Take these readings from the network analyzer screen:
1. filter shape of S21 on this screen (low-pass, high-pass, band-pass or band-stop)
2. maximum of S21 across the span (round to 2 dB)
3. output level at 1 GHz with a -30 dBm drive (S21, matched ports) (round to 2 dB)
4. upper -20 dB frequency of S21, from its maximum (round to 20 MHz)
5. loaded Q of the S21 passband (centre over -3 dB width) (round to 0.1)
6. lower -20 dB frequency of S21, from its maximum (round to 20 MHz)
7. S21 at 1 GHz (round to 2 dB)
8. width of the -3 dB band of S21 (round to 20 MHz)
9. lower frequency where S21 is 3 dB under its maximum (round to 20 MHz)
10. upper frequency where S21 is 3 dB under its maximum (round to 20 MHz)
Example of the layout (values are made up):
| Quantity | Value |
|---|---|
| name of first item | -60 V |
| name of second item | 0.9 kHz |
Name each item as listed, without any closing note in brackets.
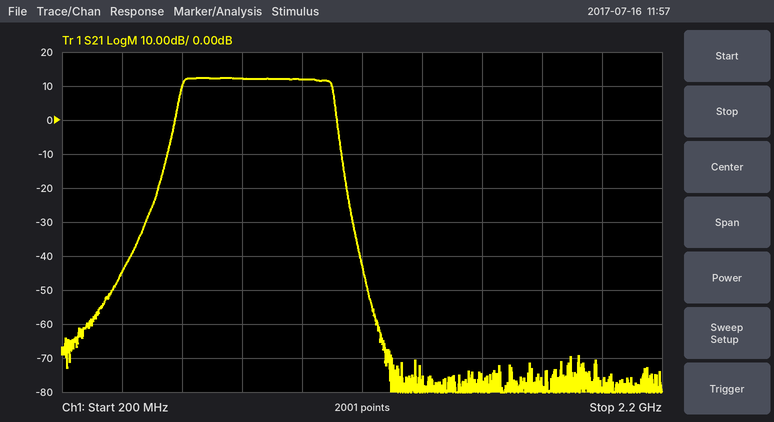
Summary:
| Quantity | Value |
|---|---|
| filter shape of S21 on this screen | band-pass |
| maximum of S21 across the span | 12 dB |
| output level at 1 GHz with a -30 dBm drive (S21, matched ports) | -18 dBm |
| upper -20 dB frequency of S21, from its maximum | 1.12 GHz |
| loaded Q of the S21 passband (centre over -3 dB width) | 1.7 |
| lower -20 dB frequency of S21, from its maximum | 560 MHz |
| S21 at 1 GHz | 12 dB |
| width of the -3 dB band of S21 | 500 MHz |
| lower frequency where S21 is 3 dB under its maximum | 600 MHz |
| upper frequency where S21 is 3 dB under its maximum | 1.10 GHz |
